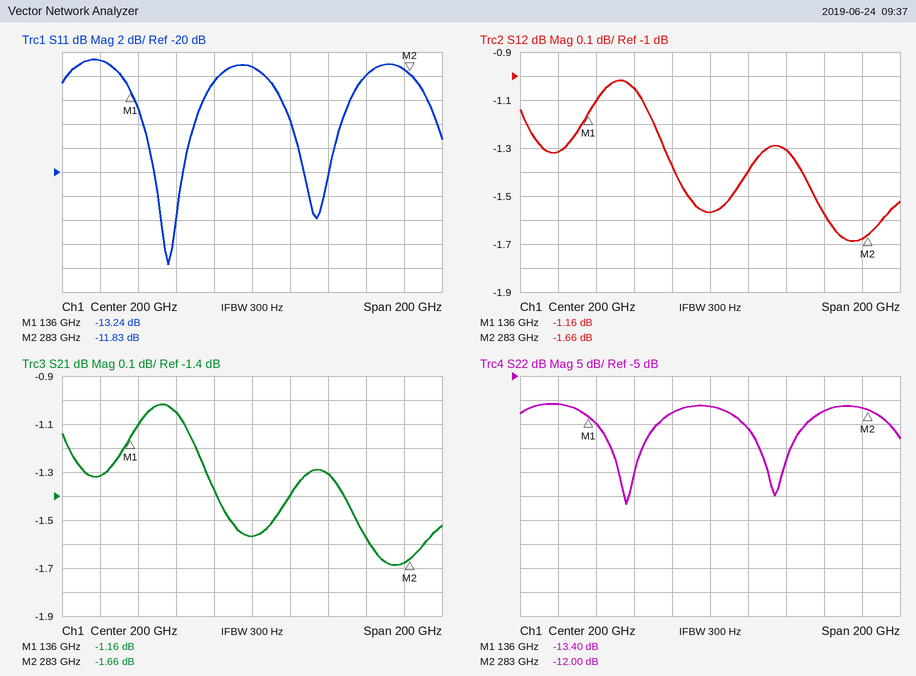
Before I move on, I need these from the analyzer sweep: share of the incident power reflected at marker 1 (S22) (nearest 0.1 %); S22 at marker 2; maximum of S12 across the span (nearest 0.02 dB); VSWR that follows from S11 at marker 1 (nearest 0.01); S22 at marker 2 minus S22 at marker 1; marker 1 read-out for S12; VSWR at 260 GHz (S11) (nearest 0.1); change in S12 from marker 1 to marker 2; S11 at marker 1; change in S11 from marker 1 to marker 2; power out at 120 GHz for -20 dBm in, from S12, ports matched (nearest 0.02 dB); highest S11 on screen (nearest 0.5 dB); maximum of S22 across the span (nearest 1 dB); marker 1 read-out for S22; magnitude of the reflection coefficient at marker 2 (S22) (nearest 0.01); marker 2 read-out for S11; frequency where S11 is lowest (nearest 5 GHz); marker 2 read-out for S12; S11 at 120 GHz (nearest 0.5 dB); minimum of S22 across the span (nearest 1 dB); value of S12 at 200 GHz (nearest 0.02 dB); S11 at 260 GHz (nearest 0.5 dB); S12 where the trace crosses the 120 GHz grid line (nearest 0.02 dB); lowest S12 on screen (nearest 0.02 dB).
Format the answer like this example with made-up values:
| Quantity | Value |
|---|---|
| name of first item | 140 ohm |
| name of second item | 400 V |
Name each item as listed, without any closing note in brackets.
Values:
| Quantity | Value |
|---|---|
| share of the incident power reflected at marker 1 (S22) | 4.6 % |
| S22 at marker 2 | -12.00 dB |
| maximum of S12 across the span | -1.02 dB |
| VSWR that follows from S11 at marker 1 | 1.56 |
| S22 at marker 2 minus S22 at marker 1 | 1.40 dB |
| marker 1 read-out for S12 | -1.16 dB |
| VSWR at 260 GHz (S11) | 1.7 |
| change in S12 from marker 1 to marker 2 | -0.50 dB |
| S11 at marker 1 | -13.24 dB |
| change in S11 from marker 1 to marker 2 | 1.41 dB |
| power out at 120 GHz for -20 dBm in, from S12, ports matched | -21.32 dBm |
| highest S11 on screen | -10.5 dB |
| maximum of S22 across the span | -11 dB |
| marker 1 read-out for S22 | -13.40 dB |
| magnitude of the reflection coefficient at marker 2 (S22) | 0.25 |
| marker 2 read-out for S11 | -11.83 dB |
| frequency where S11 is lowest | 155 GHz |
| marker 2 read-out for S12 | -1.66 dB |
| S11 at 120 GHz | -10.5 dB |
| minimum of S22 across the span | -32 dB |
| value of S12 at 200 GHz | -1.56 dB |
| S11 at 260 GHz | -12.0 dB |
| S12 where the trace crosses the 120 GHz grid line | -1.32 dB |
| lowest S12 on screen | -1.68 dB |
